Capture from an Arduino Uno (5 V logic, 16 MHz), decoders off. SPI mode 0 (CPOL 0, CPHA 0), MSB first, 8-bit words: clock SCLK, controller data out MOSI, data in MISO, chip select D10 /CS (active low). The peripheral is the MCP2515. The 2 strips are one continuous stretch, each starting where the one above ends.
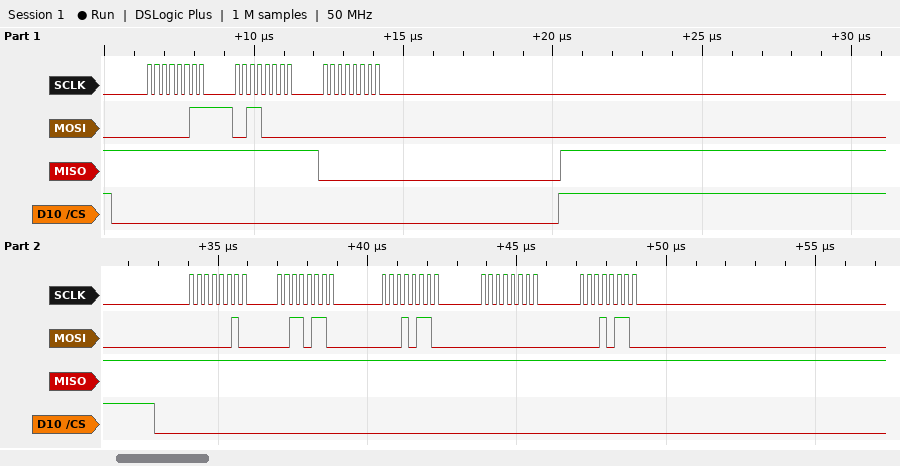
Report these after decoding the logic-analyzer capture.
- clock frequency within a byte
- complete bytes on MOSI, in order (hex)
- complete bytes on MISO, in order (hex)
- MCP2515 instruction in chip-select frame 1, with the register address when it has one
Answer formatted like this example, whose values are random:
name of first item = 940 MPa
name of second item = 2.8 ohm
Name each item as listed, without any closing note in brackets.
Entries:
clock frequency within a byte = 4 MHz
complete bytes on MOSI, in order = 03 30 00 02 36 16 00 16
complete bytes on MISO, in order = FF FF 00 FF FF FF FF FF
MCP2515 instruction in chip-select frame 1, with the register address when it has one = READ 0x30
